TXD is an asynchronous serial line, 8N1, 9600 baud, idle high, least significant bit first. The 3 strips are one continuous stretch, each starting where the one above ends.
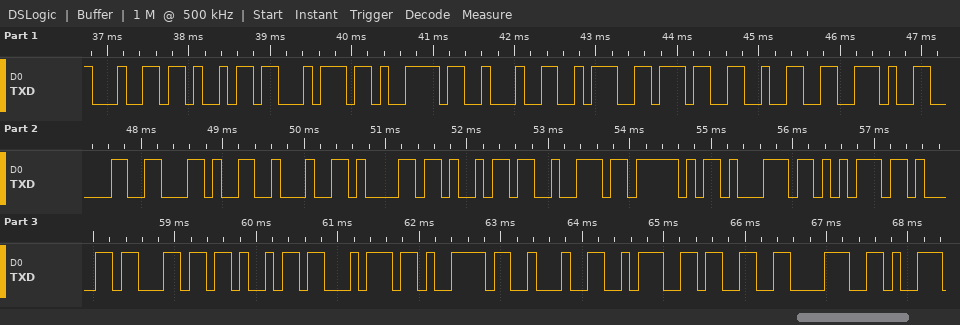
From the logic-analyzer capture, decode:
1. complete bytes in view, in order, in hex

64 69 74 79 22 3A 37 32 2E 30 2C 22 61 69 72 5F 71 75 61 6C 69 74 79 22 3A 33 38
